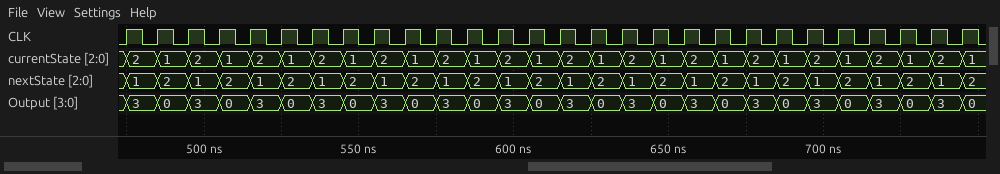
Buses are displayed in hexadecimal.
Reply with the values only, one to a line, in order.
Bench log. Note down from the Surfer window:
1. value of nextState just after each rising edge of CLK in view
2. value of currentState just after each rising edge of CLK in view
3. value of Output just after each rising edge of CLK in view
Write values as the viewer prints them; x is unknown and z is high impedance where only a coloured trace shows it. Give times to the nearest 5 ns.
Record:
1, 2, 1, 2, 1, 2, 1, 2, 1, 2, 1, 2, 1, 2, 1, 2, 1, 2, 1, 2, 1, 2, 1, 2, 1, 2, 1, 2
2, 1, 2, 1, 2, 1, 2, 1, 2, 1, 2, 1, 2, 1, 2, 1, 2, 1, 2, 1, 2, 1, 2, 1, 2, 1, 2, 1
3, 0, 3, 0, 3, 0, 3, 0, 3, 0, 3, 0, 3, 0, 3, 0, 3, 0, 3, 0, 3, 0, 3, 0, 3, 0, 3, 0
